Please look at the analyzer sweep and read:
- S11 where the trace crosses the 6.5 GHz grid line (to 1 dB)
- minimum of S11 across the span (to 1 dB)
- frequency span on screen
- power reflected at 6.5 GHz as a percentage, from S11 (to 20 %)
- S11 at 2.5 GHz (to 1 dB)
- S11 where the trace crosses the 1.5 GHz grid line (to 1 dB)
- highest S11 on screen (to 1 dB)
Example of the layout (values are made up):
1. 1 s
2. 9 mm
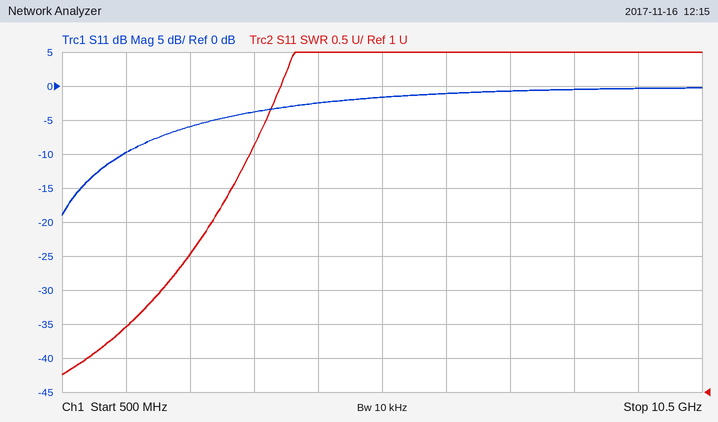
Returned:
1. -1 dB
2. -19 dB
3. 10 GHz
4. 80 %
5. -6 dB
6. -10 dB
7. 0 dB
